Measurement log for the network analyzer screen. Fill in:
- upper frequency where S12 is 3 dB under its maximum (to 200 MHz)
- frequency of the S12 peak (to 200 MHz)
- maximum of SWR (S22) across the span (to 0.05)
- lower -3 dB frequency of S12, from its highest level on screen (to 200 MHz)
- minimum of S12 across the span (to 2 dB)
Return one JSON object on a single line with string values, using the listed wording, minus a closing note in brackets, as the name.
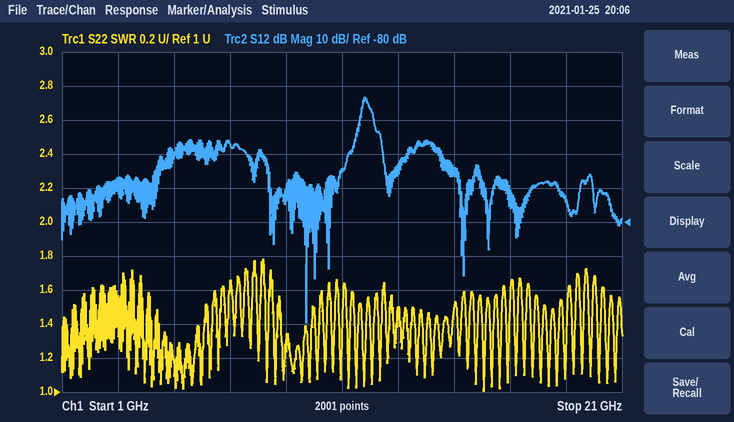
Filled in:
{"upper frequency where S12 is 3 dB under its maximum": "12.0 GHz", "frequency of the S12 peak": "11.8 GHz", "maximum of SWR (S22) across the span": "1.80", "lower -3 dB frequency of S12, from its highest level on screen": "11.8 GHz", "minimum of S12 across the span": "-110 dB"}
